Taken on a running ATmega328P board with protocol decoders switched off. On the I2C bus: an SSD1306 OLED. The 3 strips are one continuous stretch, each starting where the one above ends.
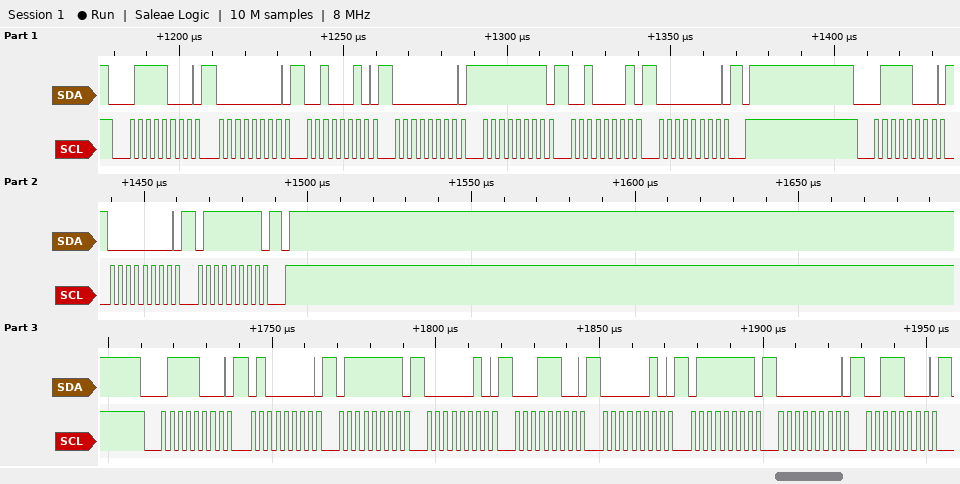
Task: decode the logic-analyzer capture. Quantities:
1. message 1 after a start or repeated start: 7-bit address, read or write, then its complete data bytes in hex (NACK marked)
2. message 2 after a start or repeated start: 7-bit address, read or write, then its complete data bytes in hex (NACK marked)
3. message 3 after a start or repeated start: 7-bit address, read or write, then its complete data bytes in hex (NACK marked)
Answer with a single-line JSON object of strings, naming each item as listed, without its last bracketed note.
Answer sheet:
{"message 1 after a start or repeated start: 7-bit address, read or write, then its complete data bytes in hex": "0x3C write: 00 22 00 FF 21 00", "message 2 after a start or repeated start: 7-bit address, read or write, then its complete data bytes in hex": "0x3C write: 00 7F", "message 3 after a start or repeated start: 7-bit address, read or write, then its complete data bytes in hex": "0x3C write: 40 7F 02 1C 02 7F 00 38"}
